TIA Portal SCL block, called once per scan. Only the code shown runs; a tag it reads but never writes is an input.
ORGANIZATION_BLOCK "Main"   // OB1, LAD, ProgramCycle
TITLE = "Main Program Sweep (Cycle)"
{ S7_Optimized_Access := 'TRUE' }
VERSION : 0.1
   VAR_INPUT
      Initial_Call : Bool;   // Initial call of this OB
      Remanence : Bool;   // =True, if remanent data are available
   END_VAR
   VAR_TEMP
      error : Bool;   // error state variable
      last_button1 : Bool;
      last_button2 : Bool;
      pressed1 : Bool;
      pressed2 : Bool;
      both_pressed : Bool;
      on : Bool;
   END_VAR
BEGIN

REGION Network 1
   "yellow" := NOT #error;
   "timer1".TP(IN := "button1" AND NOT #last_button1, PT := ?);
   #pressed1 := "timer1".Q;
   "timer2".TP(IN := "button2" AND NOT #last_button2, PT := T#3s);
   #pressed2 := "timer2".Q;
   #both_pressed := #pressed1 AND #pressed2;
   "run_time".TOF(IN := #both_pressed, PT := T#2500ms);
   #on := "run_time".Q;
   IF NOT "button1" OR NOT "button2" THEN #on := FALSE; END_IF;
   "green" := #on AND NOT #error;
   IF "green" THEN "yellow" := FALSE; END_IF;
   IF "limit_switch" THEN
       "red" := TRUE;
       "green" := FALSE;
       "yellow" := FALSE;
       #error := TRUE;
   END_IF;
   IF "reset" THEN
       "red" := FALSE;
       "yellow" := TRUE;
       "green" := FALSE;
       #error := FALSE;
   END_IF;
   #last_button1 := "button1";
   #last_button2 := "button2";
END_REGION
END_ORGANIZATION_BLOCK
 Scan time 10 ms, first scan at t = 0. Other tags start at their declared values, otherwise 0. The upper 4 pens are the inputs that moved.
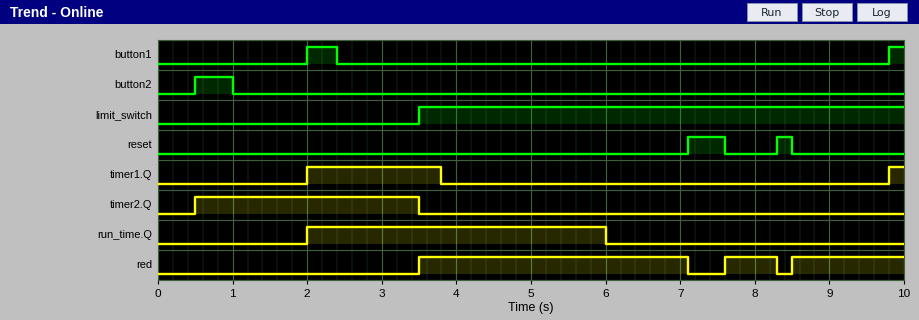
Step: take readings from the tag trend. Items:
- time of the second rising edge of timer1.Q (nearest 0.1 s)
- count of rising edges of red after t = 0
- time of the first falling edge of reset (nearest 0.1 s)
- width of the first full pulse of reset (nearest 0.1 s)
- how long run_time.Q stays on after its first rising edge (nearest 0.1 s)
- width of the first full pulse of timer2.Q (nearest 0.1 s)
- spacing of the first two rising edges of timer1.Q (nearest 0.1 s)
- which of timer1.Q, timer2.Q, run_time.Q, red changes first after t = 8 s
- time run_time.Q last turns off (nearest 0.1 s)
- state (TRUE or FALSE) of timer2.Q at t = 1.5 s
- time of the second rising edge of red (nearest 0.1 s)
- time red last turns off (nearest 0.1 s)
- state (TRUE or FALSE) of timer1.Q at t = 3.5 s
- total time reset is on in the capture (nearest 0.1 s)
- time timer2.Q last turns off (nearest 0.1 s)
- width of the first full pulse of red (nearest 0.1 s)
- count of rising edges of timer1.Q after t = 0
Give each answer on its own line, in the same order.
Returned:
9.8 s
3
7.6 s
0.5 s
4.0 s
3.0 s
7.8 s
red
6.0 s
TRUE
7.6 s
8.3 s
TRUE
0.7 s
3.5 s
3.6 s
2
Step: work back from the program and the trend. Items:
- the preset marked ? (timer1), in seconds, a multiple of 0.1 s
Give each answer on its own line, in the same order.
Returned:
1.8 s
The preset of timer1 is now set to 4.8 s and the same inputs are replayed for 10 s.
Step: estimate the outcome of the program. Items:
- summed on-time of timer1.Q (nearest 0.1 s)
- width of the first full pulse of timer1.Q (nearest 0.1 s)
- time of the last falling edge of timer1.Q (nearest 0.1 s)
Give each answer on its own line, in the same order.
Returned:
5.0 s
4.8 s
6.8 s
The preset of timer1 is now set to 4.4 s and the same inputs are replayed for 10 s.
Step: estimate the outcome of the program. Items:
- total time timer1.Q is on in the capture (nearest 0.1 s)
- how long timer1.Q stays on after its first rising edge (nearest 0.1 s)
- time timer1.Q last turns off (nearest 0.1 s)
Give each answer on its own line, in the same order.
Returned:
4.6 s
4.4 s
6.4 s
